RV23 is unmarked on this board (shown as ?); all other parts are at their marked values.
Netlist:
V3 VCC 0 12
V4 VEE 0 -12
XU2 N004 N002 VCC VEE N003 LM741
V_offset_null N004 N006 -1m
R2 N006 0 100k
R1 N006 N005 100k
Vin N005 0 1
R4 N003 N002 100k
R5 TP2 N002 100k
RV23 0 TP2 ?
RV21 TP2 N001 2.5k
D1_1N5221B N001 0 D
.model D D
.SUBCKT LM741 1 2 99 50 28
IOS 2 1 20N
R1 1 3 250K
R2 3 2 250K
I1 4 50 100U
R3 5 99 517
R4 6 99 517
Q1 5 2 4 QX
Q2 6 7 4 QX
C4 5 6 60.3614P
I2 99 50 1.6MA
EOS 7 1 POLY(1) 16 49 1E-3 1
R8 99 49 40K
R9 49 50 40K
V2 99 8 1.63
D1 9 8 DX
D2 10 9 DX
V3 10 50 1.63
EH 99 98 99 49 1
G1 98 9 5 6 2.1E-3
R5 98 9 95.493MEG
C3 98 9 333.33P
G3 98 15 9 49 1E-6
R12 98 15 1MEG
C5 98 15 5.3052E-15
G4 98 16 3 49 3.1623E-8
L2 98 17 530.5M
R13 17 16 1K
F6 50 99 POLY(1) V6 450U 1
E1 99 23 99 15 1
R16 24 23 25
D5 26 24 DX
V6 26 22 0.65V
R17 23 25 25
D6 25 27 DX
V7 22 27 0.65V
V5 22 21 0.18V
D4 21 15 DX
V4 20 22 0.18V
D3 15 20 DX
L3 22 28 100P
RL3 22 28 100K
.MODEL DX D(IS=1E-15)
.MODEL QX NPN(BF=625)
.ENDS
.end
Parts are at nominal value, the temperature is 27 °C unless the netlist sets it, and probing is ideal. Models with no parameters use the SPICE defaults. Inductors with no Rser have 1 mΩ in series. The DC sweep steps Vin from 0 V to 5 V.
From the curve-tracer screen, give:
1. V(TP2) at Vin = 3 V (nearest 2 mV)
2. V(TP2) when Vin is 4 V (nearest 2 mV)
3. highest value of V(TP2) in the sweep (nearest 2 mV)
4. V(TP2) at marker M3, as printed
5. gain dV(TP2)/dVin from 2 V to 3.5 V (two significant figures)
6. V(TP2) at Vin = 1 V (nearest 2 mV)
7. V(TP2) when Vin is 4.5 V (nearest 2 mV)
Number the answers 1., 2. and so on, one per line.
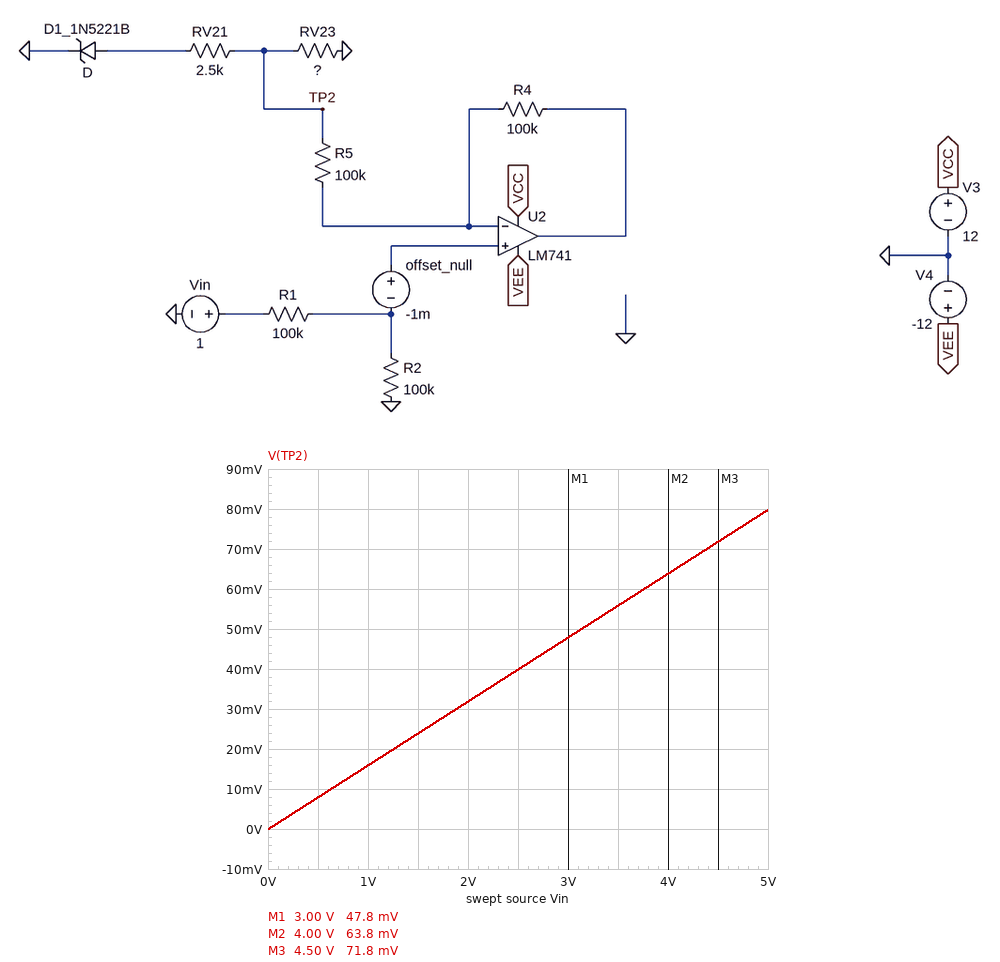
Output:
1. 48 mV
2. 64 mV
3. 80 mV
4. 71.8 mV
5. 0.016 V/V
6. 16 mV
7. 72 mV
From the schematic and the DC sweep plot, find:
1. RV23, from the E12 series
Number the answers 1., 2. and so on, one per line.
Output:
1. 3.3 kΩ
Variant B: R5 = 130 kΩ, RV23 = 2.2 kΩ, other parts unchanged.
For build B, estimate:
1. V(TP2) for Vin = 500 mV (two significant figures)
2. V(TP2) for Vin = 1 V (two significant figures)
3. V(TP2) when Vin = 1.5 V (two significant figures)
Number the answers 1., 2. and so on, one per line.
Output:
1. 4.1 mV
2. 8.3 mV
3. 12 mV
